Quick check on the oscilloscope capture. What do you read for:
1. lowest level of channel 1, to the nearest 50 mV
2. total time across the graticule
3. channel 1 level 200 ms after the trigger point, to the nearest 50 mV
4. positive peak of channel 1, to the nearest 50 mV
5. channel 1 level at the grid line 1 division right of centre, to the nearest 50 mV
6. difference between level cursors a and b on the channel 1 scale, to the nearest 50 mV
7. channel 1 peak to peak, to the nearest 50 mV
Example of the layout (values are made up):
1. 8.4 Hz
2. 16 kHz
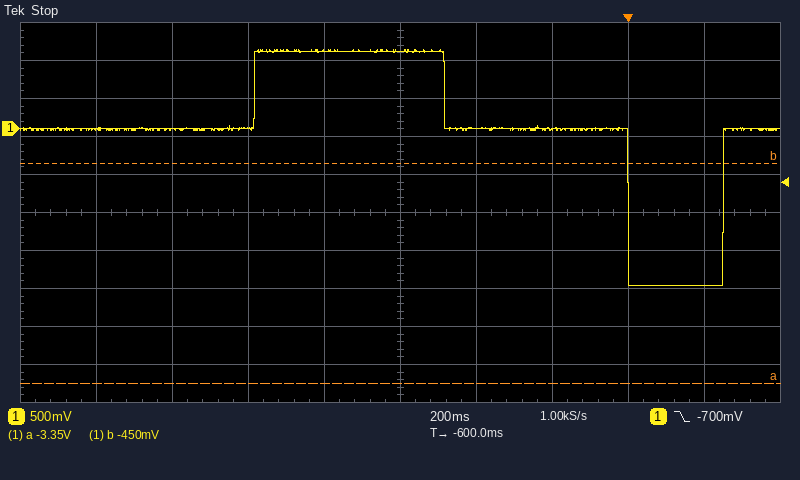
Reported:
1. -2.05 V
2. 2 s
3. -2.05 V
4. 1.05 V
5. 0 mV
6. 2.90 V
7. 3.10 V
